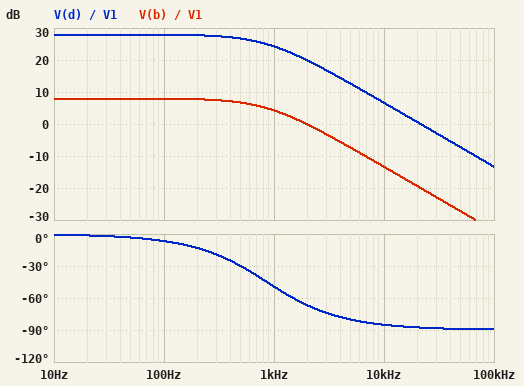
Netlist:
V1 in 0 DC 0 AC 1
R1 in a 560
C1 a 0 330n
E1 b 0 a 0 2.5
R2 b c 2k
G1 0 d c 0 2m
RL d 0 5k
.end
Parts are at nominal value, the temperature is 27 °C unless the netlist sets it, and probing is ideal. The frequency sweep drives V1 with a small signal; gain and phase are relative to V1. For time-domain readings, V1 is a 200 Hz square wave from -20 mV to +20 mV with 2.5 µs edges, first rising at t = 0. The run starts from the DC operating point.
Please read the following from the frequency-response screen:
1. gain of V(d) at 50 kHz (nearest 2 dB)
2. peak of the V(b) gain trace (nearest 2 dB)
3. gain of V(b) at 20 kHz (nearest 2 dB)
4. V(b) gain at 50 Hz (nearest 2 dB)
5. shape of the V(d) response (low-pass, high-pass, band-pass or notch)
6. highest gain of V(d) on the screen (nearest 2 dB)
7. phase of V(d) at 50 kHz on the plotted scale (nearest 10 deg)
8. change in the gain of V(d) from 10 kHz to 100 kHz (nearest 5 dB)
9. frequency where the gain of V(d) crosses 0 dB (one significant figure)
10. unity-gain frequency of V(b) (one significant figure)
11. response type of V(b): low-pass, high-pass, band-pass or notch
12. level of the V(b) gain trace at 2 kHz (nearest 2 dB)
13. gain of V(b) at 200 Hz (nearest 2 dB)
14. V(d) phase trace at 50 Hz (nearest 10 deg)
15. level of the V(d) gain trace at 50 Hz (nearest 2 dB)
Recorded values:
-8 dB
8 dB
-20 dB
8 dB
low-pass
28 dB
-90 deg
-20 dB
20 kHz
2 kHz
low-pass
0 dB
8 dB
0 deg
28 dB
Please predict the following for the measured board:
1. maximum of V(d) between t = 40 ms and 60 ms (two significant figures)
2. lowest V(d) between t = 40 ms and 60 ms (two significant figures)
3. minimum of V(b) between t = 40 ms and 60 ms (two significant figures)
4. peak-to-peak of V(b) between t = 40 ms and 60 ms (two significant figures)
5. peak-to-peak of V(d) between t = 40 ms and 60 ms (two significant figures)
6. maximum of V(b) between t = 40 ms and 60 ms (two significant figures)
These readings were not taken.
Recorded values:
500 mV
-500 mV
-50 mV
100 mV
1.0 V
50 mV
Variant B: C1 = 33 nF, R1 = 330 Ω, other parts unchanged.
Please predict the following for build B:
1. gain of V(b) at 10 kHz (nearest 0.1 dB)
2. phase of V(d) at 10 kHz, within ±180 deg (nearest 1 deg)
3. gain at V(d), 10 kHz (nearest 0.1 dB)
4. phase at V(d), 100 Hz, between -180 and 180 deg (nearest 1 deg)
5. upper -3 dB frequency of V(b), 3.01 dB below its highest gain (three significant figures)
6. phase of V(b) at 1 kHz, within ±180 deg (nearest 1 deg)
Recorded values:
6.3 dB
-34 deg
26.3 dB
0 deg
14.6 kHz
-4 deg
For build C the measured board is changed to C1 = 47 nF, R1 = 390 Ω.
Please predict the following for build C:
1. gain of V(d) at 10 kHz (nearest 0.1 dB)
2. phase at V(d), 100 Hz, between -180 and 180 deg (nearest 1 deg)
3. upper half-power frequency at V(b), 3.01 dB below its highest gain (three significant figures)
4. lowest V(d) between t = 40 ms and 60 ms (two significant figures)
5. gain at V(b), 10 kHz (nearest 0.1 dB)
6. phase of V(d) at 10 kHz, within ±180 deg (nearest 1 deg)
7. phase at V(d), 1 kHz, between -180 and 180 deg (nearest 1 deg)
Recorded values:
24.3 dB
-1 deg
8.68 kHz
-500 mV
4.3 dB
-49 deg
-7 deg
